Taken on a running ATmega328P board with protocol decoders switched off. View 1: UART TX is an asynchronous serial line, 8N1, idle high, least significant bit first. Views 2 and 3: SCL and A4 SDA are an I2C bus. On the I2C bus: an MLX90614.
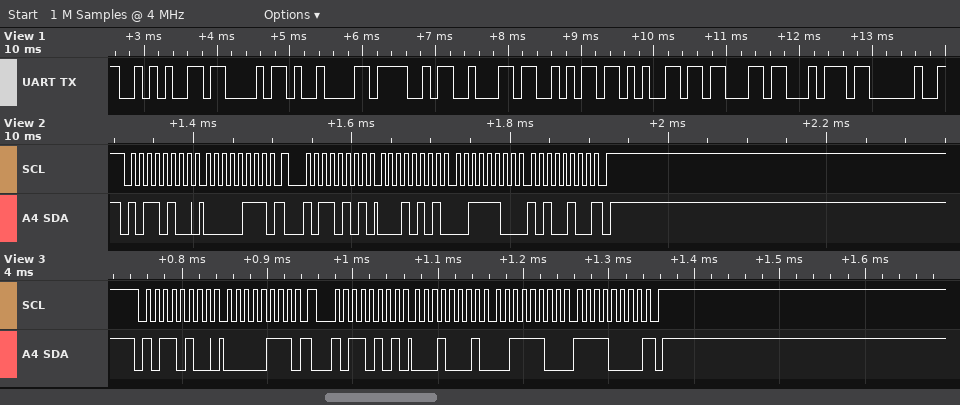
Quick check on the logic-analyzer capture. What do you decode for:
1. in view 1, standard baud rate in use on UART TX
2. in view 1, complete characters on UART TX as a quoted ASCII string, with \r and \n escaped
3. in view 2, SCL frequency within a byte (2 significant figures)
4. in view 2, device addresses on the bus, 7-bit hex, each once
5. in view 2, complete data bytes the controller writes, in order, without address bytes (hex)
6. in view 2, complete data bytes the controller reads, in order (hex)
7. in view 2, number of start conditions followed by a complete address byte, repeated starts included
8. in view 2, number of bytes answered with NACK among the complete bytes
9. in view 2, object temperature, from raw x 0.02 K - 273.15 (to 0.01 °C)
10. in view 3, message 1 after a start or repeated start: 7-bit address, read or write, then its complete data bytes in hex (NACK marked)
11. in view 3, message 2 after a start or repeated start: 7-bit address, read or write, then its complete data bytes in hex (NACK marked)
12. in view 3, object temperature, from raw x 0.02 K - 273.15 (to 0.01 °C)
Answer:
9600 baud
"*C\tObject "
100 kHz
0x5A
07
15 3C A4
2
1
34.47 °C
0x5A write: 07
0x5A read: 11 3C F0 NACK
34.39 °C
